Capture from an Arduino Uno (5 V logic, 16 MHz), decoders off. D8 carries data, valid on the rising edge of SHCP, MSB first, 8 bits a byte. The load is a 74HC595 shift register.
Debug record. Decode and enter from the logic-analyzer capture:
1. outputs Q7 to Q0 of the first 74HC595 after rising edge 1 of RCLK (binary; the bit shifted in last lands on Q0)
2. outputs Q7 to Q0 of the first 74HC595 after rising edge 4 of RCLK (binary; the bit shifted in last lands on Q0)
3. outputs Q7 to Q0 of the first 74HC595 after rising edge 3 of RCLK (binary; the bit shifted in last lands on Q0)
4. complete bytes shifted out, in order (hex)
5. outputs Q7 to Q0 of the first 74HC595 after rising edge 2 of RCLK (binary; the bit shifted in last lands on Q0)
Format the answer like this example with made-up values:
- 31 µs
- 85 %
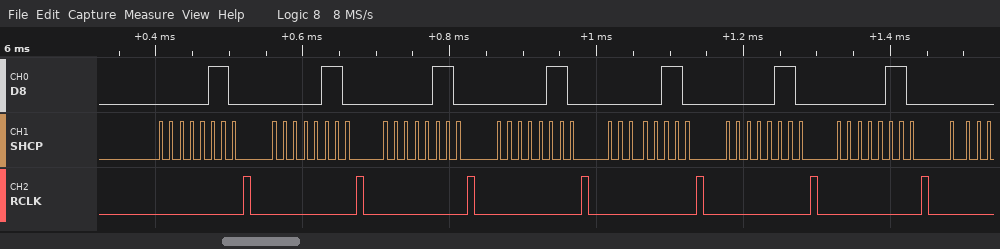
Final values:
- 00000110
- 00000110
- 00000110
- 06 06 06 06 06 06 06
- 00000110
